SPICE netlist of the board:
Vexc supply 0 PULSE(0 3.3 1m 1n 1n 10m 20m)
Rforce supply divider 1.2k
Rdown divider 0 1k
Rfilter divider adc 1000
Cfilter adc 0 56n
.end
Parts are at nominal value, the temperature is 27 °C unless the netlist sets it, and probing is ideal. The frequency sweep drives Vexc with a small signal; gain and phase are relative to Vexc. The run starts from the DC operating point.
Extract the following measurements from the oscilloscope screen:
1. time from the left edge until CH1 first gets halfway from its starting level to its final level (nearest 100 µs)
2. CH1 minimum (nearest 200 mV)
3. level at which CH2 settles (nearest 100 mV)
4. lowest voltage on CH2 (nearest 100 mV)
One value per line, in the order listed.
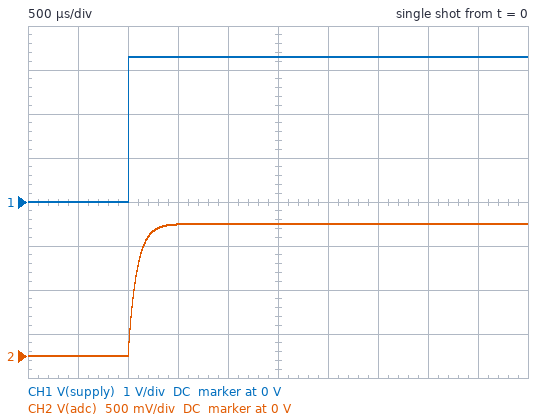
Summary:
1.0 ms
0 V
1.5 V
0 V
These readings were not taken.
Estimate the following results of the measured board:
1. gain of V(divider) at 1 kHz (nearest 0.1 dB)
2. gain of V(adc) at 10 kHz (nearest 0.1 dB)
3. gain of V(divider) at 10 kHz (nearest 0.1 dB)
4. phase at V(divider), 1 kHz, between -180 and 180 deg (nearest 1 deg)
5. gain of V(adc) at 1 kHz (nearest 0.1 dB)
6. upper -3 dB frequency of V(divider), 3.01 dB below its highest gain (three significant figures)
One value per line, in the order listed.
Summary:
-7.5 dB
-21.7 dB
-10.4 dB
-9 deg
-8.0 dB
4.56 kHz
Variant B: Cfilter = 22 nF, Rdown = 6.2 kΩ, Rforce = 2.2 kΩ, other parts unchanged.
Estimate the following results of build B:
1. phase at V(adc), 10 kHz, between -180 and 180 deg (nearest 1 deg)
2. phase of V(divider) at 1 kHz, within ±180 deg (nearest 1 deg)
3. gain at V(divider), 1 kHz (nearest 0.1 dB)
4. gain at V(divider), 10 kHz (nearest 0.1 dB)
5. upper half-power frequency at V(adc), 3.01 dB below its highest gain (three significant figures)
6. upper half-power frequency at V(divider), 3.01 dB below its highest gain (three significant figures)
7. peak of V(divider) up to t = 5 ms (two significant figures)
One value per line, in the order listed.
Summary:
-75 deg
-12 deg
-3.1 dB
-9.5 dB
2.76 kHz
3.27 kHz
2.4 V
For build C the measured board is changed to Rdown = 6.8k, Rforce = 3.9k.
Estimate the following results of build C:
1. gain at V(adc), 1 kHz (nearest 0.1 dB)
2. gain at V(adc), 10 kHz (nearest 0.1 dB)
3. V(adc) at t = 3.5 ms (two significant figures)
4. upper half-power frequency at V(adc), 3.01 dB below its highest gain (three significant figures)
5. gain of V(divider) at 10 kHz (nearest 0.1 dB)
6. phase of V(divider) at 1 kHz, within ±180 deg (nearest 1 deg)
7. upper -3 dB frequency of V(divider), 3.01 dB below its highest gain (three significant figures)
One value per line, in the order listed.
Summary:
-7.9 dB
-25.7 dB
2.1 V
817 Hz
-14.5 dB
-31 deg
894 Hz
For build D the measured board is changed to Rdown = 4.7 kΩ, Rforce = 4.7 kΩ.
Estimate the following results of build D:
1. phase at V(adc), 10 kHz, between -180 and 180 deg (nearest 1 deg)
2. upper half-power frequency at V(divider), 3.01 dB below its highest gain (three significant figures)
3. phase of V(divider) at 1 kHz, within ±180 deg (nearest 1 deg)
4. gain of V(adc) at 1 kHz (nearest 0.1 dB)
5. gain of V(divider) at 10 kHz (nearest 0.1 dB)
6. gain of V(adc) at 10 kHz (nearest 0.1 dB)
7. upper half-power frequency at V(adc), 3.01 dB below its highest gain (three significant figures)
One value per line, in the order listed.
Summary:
-85 deg
936 Hz
-30 deg
-9.8 dB
-16.2 dB
-27.5 dB
848 Hz
